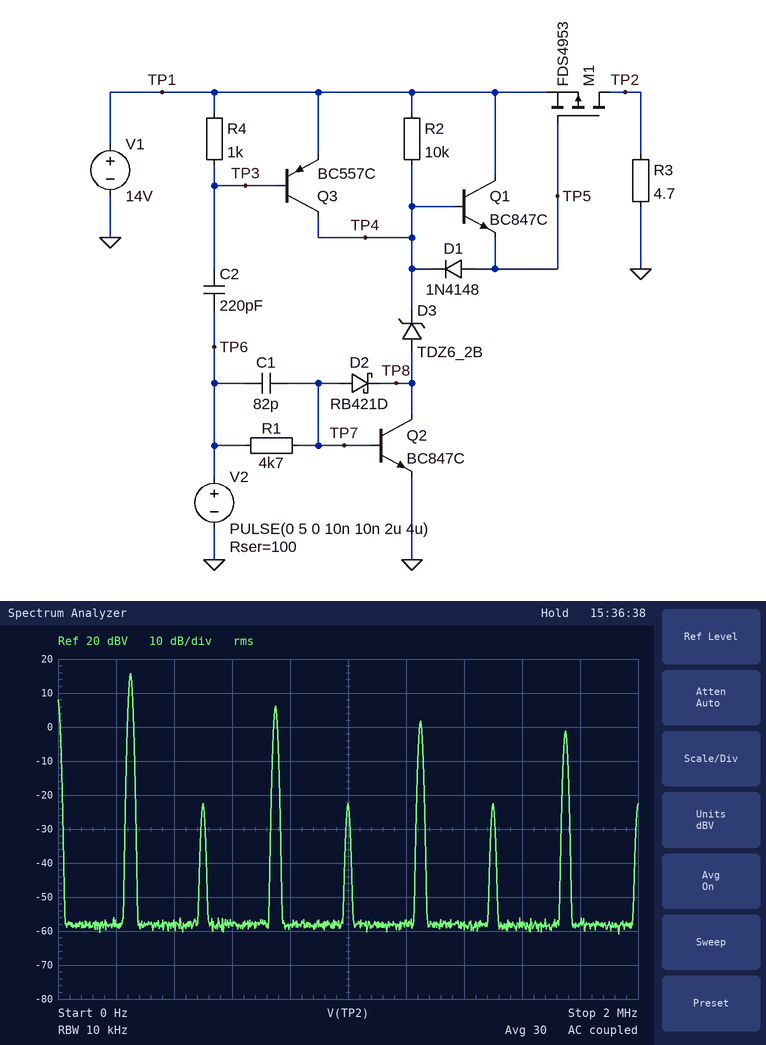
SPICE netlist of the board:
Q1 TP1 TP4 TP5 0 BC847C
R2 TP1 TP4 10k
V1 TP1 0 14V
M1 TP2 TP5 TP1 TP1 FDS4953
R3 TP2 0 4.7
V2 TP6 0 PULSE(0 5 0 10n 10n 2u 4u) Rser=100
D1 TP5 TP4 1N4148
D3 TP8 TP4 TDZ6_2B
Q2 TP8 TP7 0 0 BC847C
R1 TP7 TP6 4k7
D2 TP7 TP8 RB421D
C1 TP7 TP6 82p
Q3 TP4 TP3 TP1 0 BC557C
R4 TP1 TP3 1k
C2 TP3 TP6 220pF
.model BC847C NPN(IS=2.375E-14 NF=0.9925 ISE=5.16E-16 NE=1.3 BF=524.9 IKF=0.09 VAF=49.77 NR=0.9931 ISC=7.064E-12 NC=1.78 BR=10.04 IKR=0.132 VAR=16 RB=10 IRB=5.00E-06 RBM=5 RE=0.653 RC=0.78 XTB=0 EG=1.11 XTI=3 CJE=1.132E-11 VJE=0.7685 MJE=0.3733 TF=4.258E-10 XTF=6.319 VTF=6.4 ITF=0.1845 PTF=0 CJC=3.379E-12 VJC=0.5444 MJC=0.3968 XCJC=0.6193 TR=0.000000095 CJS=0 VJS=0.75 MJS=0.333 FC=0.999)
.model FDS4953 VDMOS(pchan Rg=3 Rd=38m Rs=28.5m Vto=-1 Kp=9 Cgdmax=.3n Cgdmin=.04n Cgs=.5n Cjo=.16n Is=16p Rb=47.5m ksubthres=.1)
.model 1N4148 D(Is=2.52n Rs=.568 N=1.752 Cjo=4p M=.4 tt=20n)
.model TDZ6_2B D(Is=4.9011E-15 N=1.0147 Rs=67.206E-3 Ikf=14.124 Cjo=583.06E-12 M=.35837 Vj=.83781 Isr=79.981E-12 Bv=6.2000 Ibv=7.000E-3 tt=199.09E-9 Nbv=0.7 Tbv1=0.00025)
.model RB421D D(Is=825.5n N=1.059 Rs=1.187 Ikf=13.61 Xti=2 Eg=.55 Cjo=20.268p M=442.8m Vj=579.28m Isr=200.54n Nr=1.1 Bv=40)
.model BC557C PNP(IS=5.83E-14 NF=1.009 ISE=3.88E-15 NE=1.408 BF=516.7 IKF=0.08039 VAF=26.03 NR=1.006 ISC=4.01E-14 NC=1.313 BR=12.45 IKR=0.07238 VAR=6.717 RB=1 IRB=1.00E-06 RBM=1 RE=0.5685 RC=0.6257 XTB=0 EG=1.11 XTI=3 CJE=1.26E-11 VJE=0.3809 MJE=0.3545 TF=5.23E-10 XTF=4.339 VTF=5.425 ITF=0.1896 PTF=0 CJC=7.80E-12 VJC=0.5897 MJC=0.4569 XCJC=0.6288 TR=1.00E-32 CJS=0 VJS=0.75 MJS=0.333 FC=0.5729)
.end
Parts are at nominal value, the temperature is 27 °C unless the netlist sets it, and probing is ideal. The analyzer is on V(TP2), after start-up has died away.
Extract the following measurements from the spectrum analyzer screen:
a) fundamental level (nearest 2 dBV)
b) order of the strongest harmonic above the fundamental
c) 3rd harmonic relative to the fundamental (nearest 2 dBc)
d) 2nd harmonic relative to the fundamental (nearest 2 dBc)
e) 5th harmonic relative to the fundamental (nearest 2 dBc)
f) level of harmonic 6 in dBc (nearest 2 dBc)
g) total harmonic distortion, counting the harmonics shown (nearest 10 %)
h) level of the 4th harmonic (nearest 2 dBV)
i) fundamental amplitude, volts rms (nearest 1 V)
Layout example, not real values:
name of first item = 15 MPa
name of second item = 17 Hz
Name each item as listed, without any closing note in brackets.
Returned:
fundamental level = 16 dBV
order of the strongest harmonic above the fundamental = 3
3rd harmonic relative to the fundamental = -10 dBc
2nd harmonic relative to the fundamental = -38 dBc
5th harmonic relative to the fundamental = -14 dBc
level of harmonic 6 in dBc = -38 dBc
total harmonic distortion, counting the harmonics shown = 40 %
level of the 4th harmonic = -22 dBV
fundamental amplitude, volts rms = 6 V
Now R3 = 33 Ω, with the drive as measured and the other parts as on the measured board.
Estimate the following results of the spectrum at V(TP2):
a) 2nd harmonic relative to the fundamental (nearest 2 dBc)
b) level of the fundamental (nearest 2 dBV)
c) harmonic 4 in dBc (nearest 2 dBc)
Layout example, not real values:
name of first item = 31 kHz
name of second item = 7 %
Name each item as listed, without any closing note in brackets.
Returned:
2nd harmonic relative to the fundamental = -36 dBc
level of the fundamental = 16 dBV
harmonic 4 in dBc = -36 dBc
